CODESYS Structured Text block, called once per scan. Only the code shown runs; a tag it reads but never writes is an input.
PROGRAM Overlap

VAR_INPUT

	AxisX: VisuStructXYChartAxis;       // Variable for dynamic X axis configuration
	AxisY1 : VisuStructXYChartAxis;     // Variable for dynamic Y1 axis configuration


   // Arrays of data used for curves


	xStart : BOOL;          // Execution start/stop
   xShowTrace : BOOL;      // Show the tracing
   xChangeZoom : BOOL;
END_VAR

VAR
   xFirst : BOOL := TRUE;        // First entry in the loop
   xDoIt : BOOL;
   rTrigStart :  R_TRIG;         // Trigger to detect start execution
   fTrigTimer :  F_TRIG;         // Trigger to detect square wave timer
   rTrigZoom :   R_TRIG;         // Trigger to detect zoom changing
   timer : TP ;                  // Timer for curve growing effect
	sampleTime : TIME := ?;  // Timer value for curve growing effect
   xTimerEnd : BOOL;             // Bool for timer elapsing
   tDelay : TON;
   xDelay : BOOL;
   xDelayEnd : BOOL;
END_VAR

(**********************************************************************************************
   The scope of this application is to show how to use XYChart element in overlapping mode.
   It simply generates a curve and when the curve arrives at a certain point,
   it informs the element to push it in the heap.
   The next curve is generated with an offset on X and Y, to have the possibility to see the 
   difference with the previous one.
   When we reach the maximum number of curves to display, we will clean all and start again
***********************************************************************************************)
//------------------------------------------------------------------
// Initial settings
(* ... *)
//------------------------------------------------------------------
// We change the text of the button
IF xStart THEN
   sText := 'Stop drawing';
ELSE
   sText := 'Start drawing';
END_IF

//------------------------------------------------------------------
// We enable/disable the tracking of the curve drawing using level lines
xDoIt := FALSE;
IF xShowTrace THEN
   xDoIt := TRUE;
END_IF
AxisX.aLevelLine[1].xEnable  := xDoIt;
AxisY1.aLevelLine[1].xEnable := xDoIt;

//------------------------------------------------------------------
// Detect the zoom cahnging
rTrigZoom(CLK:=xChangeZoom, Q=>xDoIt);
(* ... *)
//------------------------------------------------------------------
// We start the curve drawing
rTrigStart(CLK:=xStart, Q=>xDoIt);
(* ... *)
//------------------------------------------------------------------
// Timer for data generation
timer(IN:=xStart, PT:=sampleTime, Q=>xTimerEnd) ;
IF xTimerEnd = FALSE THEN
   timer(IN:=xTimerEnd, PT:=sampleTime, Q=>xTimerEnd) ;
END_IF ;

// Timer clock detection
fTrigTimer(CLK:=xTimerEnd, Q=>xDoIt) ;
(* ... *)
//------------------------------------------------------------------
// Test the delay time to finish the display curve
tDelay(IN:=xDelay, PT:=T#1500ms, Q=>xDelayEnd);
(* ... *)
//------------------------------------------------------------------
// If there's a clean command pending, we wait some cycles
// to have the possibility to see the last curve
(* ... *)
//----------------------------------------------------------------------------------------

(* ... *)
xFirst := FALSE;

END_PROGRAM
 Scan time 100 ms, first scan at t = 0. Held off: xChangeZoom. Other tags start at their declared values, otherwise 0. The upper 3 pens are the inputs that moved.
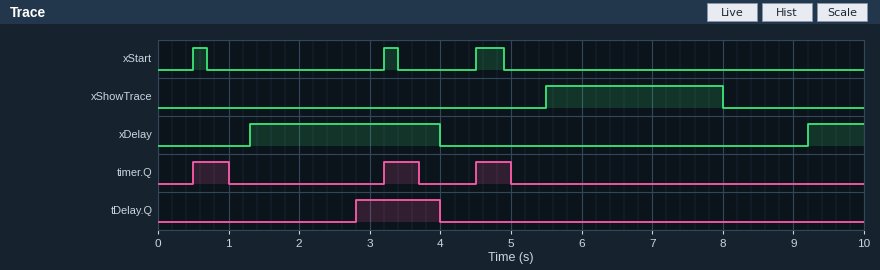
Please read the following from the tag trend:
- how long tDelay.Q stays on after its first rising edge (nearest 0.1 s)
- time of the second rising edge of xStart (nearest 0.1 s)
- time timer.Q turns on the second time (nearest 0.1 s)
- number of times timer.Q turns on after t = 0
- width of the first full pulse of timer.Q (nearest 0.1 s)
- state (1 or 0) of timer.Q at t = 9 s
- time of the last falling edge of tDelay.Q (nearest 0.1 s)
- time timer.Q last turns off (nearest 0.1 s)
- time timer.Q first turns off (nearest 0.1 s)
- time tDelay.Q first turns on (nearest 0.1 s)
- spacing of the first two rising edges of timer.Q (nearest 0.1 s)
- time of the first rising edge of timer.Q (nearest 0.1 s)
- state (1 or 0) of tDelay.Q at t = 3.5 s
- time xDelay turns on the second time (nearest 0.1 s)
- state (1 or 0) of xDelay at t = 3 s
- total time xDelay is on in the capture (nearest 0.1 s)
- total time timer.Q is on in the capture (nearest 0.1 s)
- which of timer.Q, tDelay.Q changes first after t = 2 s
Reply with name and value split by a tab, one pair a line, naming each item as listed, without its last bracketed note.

how long tDelay.Q stays on after its first rising edge	1.2 s
time of the second rising edge of xStart	3.2 s
time timer.Q turns on the second time	3.2 s
number of times timer.Q turns on after t = 0	3
width of the first full pulse of timer.Q	0.5 s
state (1 or 0) of timer.Q at t = 9 s	0
time of the last falling edge of tDelay.Q	4.0 s
time timer.Q last turns off	5.0 s
time timer.Q first turns off	1.0 s
time tDelay.Q first turns on	2.8 s
spacing of the first two rising edges of timer.Q	2.7 s
time of the first rising edge of timer.Q	0.5 s
state (1 or 0) of tDelay.Q at t = 3.5 s	1
time xDelay turns on the second time	9.2 s
state (1 or 0) of xDelay at t = 3 s	1
total time xDelay is on in the capture	3.5 s
total time timer.Q is on in the capture	1.5 s
which of timer.Q, tDelay.Q changes first after t = 2 s	tDelay.Q
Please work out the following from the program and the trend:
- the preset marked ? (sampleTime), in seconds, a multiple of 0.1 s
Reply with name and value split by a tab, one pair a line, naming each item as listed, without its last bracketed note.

the preset marked ? (sampleTime), in seconds, a multiple of 0.1 s	0.5 s
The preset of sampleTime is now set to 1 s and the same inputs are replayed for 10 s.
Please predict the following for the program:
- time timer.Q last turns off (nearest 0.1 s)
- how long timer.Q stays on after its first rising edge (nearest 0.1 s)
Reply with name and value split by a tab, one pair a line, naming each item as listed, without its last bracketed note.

time timer.Q last turns off	5.5 s
how long timer.Q stays on after its first rising edge	1.0 s
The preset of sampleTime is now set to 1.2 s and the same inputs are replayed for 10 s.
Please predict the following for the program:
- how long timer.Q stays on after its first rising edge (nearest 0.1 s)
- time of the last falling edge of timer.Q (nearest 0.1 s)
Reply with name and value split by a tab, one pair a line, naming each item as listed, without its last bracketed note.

how long timer.Q stays on after its first rising edge	1.2 s
time of the last falling edge of timer.Q	5.7 s
